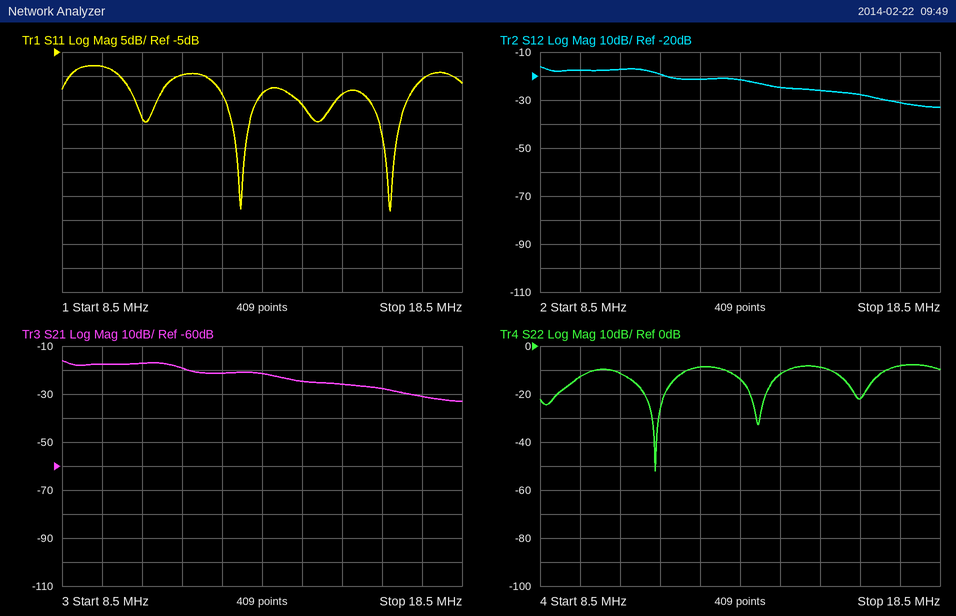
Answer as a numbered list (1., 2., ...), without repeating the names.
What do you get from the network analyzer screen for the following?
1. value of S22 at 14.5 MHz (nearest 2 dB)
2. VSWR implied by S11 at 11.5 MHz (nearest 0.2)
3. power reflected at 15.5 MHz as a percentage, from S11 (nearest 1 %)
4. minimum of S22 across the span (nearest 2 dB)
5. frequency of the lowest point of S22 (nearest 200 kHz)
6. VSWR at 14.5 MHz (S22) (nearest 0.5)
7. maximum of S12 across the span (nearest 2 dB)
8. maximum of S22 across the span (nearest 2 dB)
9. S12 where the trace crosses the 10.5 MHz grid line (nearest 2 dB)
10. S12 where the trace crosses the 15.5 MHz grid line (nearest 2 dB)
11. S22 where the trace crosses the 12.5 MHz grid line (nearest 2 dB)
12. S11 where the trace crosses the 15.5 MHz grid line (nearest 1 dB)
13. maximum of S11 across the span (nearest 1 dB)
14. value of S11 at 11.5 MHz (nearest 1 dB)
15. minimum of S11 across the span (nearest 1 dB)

1. -12 dB
2. 2.0
3. 4 %
4. -52 dB
5. 11.4 MHz
6. 1.5
7. -16 dB
8. -8 dB
9. -18 dB
10. -26 dB
11. -8 dB
12. -14 dB
13. -8 dB
14. -10 dB
15. -38 dB
